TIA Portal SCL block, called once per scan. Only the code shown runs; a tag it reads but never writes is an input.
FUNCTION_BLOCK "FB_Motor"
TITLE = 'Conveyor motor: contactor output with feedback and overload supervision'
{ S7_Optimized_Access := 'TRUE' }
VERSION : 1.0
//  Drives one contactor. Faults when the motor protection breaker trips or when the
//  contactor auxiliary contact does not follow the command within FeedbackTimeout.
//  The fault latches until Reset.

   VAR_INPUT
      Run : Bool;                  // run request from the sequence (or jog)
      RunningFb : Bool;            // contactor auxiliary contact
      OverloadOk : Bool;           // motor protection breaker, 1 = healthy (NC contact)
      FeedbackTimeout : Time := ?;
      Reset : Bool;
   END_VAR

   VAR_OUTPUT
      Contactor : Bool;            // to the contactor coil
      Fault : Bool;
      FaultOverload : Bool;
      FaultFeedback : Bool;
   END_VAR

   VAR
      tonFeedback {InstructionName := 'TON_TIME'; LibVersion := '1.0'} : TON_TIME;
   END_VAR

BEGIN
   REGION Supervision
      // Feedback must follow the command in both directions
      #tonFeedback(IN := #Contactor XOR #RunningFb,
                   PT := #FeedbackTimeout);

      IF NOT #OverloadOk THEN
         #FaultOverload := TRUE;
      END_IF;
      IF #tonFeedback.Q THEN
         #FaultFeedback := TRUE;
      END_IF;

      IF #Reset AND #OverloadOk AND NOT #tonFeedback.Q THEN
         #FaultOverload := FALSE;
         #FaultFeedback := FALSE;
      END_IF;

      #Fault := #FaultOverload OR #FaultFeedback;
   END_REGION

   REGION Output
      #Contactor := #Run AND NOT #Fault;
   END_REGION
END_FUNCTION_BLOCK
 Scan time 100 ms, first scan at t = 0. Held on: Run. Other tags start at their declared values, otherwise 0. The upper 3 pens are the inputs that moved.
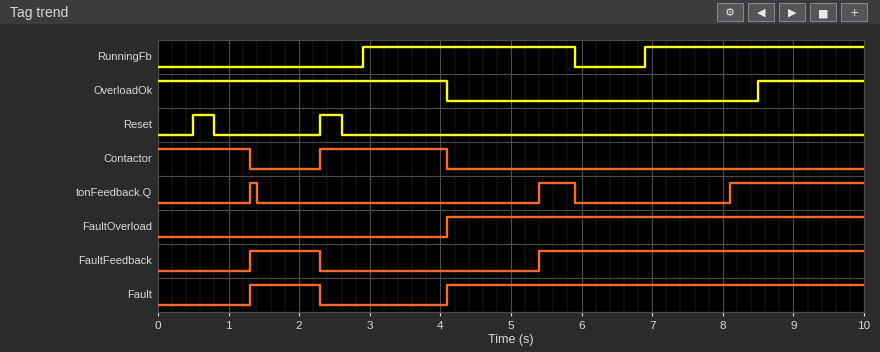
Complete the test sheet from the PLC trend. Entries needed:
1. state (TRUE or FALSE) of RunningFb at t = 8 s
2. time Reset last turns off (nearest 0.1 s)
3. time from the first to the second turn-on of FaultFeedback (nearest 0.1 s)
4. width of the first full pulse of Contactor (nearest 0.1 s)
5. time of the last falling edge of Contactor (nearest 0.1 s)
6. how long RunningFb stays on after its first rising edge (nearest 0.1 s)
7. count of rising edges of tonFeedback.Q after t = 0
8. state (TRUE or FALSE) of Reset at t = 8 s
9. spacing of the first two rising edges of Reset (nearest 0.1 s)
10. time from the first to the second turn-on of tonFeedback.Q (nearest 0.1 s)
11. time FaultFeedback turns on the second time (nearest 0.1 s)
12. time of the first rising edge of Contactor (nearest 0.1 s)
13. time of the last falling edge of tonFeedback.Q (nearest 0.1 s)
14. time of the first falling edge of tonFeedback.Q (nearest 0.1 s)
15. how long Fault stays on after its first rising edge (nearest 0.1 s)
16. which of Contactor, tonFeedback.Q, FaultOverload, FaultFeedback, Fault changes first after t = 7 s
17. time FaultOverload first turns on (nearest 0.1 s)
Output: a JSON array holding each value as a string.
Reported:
["TRUE", "2.6 s", "4.1 s", "1.8 s", "4.1 s", "3.0 s", "3", "FALSE", "1.8 s", "4.1 s", "5.4 s", "2.3 s", "5.9 s", "1.4 s", "1.0 s", "tonFeedback.Q", "4.1 s"]
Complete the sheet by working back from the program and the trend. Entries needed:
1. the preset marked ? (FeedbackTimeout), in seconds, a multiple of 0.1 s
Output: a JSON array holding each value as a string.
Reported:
["1.2 s"]
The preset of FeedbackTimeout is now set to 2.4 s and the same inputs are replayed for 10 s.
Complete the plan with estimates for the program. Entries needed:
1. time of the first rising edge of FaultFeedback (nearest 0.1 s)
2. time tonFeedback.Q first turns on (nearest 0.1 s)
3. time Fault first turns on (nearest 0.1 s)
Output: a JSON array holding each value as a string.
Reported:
["2.5 s", "2.5 s", "2.5 s"]
